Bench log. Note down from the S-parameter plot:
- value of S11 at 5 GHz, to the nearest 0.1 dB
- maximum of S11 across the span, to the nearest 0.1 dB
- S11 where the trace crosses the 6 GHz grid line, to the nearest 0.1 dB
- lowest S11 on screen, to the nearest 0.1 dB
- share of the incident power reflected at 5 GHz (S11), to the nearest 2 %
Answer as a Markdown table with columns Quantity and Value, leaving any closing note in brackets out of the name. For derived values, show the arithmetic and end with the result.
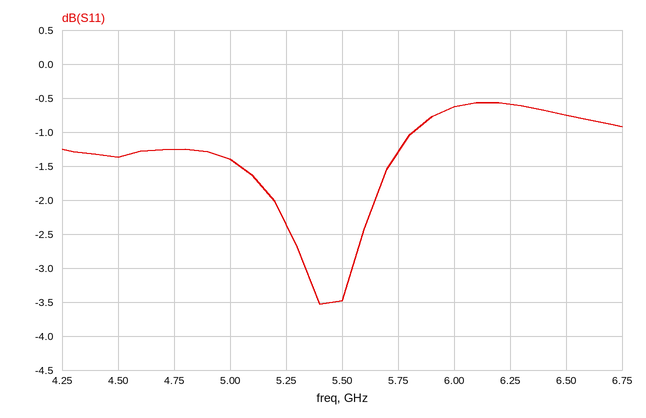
| Quantity | Value |
|---|---|
| value of S11 at 5 GHz, to the nearest 0.1 dB | -1.4 dB |
| maximum of S11 across the span, to the nearest 0.1 dB | -0.6 dB |
| S11 where the trace crosses the 6 GHz grid line, to the nearest 0.1 dB | -0.6 dB |
| lowest S11 on screen, to the nearest 0.1 dB | -3.5 dB |
| share of the incident power reflected at 5 GHz (S11), to the nearest 2 % | 10^(-1.4/10) ≈ 72 % |
